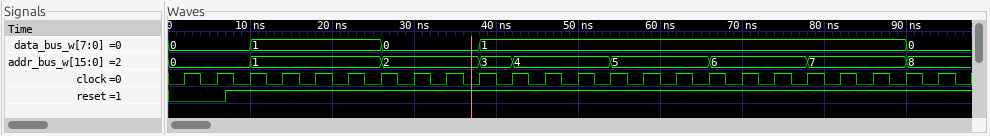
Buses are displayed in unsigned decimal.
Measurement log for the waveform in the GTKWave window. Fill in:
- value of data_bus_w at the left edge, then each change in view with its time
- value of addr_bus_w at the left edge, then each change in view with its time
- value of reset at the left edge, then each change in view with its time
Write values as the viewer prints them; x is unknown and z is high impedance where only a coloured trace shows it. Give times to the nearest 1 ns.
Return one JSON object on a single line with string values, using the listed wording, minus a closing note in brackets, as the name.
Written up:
{"value of data_bus_w at the left edge, then each change in view with its time": "0, 1 at 10 ns, 0 at 26 ns, 1 at 38 ns, 0 at 90 ns", "value of addr_bus_w at the left edge, then each change in view with its time": "0, 1 at 10 ns, 2 at 26 ns, 3 at 38 ns, 4 at 42 ns, 5 at 54 ns, 6 at 66 ns, 7 at 78 ns, 8 at 90 ns", "value of reset at the left edge, then each change in view with its time": "0, 1 at 7 ns"}
